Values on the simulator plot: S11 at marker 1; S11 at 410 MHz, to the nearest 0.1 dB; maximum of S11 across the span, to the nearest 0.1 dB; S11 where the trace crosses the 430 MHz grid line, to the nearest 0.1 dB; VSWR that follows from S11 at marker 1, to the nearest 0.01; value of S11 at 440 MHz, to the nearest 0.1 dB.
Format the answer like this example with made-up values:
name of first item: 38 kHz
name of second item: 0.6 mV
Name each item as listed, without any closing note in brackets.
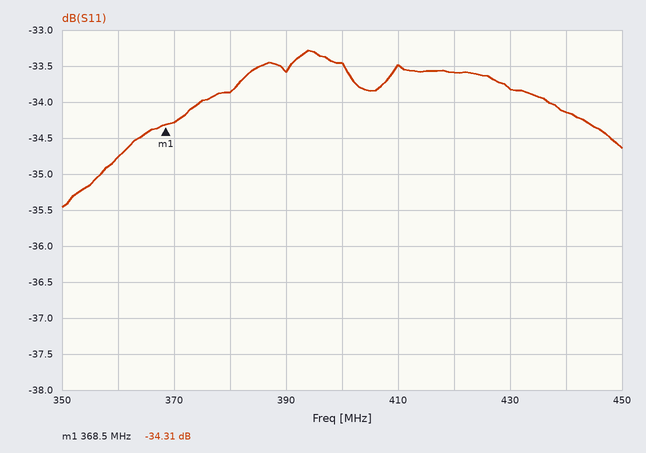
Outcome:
S11 at marker 1: -34.31 dB
S11 at 410 MHz, to the nearest 0.1 dB: -33.5 dB
maximum of S11 across the span, to the nearest 0.1 dB: -33.3 dB
S11 where the trace crosses the 430 MHz grid line, to the nearest 0.1 dB: -33.8 dB
VSWR that follows from S11 at marker 1, to the nearest 0.01: 1.04
value of S11 at 440 MHz, to the nearest 0.1 dB: -34.1 dB
